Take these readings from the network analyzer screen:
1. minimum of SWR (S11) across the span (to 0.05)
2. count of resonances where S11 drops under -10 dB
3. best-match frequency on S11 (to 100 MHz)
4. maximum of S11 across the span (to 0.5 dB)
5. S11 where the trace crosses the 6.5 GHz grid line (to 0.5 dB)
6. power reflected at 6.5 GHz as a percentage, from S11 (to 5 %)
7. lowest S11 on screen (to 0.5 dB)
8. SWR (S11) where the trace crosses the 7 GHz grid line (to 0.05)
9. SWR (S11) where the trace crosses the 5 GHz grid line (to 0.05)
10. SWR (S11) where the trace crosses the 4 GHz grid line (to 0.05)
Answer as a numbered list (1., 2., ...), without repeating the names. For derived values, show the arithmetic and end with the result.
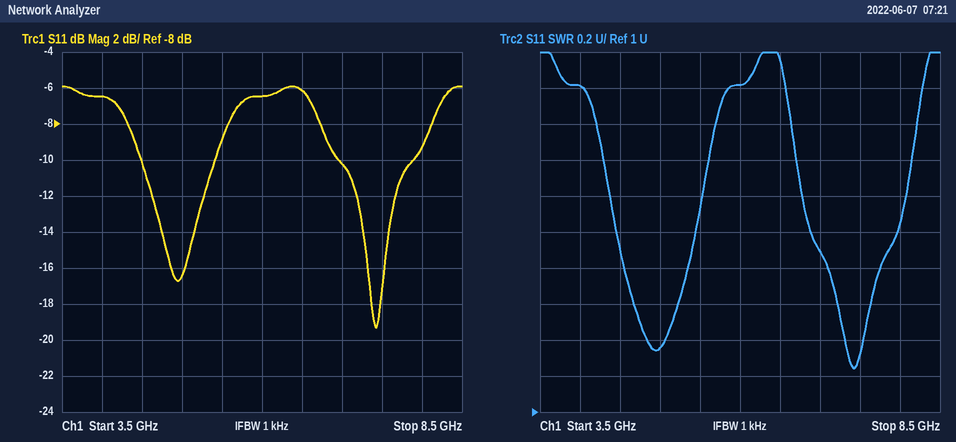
1. 1.25
2. 2
3. 7.4 GHz
4. -6.0 dB
5. -6.0 dB
6. 10^(-6/10) ≈ 25 %
7. -19.5 dB
8. 1.90
9. 1.35
10. 2.80
